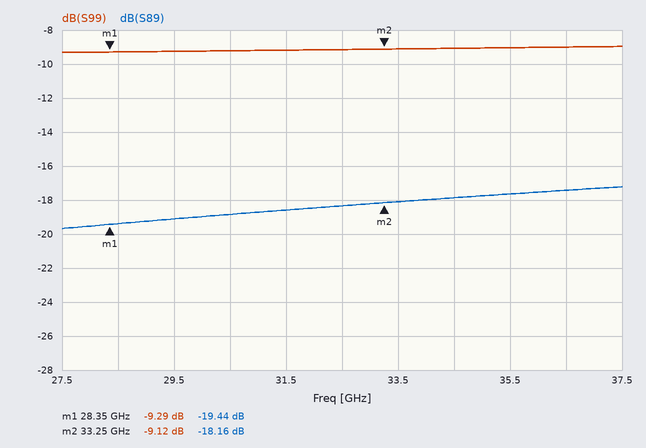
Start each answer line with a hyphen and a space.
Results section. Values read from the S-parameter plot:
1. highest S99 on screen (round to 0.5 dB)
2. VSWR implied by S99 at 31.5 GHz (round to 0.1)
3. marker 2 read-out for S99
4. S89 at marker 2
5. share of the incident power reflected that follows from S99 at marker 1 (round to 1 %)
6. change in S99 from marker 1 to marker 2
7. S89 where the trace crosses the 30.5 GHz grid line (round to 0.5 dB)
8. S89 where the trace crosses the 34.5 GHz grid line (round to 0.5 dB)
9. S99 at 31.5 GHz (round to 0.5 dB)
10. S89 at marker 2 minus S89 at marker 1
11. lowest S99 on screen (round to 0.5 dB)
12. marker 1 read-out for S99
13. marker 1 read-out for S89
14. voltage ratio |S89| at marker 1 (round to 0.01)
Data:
- -9.0 dB
- 2.1
- -9.12 dB
- -18.16 dB
- 12 %
- 0.17 dB
- -19.0 dB
- -18.0 dB
- -9.0 dB
- 1.28 dB
- -9.5 dB
- -9.29 dB
- -19.44 dB
- 0.11
